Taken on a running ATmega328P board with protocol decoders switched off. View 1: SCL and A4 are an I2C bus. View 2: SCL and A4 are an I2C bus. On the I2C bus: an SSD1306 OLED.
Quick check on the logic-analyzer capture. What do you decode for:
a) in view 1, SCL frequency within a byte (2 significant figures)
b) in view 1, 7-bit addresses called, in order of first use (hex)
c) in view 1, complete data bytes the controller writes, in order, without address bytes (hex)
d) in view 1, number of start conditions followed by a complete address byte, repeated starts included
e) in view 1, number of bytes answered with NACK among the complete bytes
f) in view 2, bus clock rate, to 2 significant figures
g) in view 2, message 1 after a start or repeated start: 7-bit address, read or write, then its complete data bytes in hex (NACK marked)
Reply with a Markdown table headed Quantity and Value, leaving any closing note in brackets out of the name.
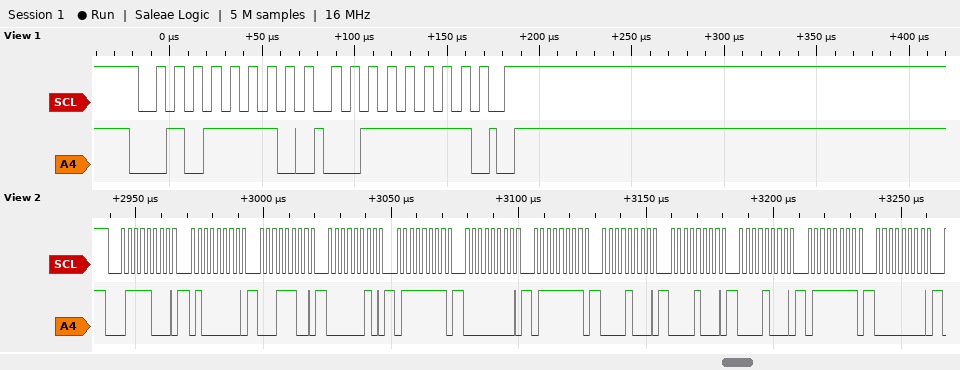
| Quantity | Value |
|---|---|
| in view 1, SCL frequency within a byte | 100 kHz |
| in view 1, 7-bit addresses called, in order of first use | 0x2F |
| in view 1, complete data bytes the controller writes, in order, without address bytes | 3F |
| in view 1, number of start conditions followed by a complete address byte, repeated starts included | 1 |
| in view 1, number of bytes answered with NACK among the complete bytes | 0 |
| in view 2, bus clock rate, to 2 significant figures | 400 kHz |
| in view 2, message 1 after a start or repeated start: 7-bit address, read or write, then its complete data bytes in hex | 0x3C write: 40 1C 02 7F 00 7F 08 08 08 7F 00 |
